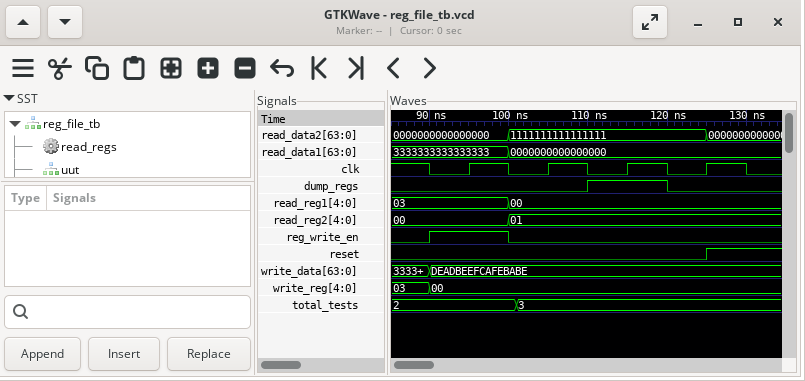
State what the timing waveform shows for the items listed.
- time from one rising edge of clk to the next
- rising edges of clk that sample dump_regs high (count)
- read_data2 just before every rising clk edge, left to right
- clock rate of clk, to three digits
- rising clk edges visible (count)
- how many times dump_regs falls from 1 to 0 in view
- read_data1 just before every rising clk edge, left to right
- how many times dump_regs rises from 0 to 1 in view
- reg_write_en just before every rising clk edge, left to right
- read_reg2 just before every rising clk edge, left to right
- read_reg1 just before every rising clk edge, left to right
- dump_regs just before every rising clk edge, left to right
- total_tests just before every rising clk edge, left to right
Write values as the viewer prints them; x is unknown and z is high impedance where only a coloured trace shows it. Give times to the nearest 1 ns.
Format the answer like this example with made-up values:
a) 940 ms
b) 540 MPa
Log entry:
a) 10 ns
b) 1
c) 0000000000000000, 1111111111111111, 1111111111111111, 1111111111111111
d) 100 MHz
e) 4
f) 1
g) 3333333333333333, 0000000000000000, 0000000000000000, 0000000000000000
h) 1
i) 1 0 0 0
j) 00, 01, 01, 01
k) 03, 00, 00, 00
l) 0 0 1 0
m) 2, 3, 3, 3
